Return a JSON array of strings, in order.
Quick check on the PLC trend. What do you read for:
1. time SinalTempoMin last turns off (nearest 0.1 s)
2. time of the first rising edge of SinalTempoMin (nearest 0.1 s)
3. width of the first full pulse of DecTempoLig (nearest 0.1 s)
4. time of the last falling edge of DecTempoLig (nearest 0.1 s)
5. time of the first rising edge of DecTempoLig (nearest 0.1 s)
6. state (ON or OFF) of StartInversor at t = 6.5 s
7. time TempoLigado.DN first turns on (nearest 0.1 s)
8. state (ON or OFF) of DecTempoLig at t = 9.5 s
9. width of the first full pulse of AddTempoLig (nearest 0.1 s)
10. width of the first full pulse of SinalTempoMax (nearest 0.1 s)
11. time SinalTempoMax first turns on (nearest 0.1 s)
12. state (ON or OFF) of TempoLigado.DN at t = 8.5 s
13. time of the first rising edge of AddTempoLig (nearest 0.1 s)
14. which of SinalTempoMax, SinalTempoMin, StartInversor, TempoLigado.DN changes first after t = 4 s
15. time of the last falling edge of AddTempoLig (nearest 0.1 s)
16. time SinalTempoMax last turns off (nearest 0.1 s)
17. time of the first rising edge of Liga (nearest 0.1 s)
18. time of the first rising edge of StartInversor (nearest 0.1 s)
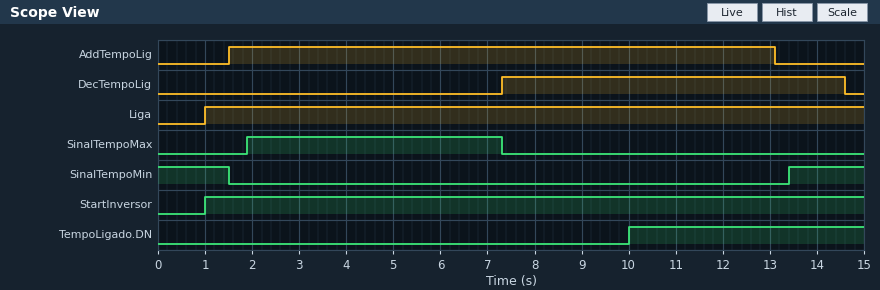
["1.5 s", "13.4 s", "7.3 s", "14.6 s", "7.3 s", "ON", "10.0 s", "ON", "11.6 s", "5.4 s", "1.9 s", "OFF", "1.5 s", "SinalTempoMax", "13.1 s", "7.3 s", "1.0 s", "1.0 s"]
